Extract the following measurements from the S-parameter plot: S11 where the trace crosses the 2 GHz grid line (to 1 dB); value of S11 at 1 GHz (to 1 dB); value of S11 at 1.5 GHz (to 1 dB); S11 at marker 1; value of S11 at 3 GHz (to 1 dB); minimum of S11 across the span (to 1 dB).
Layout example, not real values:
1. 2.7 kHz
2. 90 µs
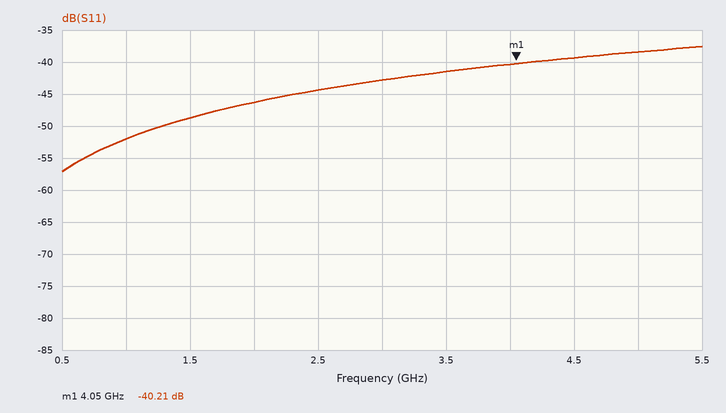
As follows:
1. -46 dB
2. -52 dB
3. -49 dB
4. -40.21 dB
5. -43 dB
6. -57 dB
